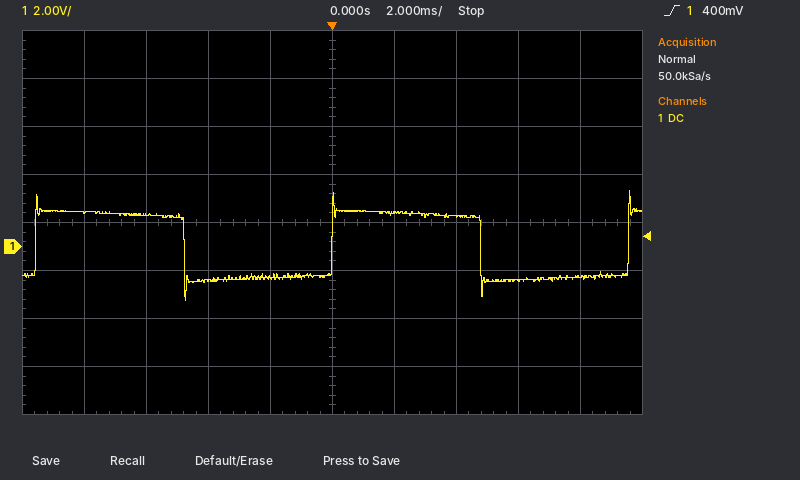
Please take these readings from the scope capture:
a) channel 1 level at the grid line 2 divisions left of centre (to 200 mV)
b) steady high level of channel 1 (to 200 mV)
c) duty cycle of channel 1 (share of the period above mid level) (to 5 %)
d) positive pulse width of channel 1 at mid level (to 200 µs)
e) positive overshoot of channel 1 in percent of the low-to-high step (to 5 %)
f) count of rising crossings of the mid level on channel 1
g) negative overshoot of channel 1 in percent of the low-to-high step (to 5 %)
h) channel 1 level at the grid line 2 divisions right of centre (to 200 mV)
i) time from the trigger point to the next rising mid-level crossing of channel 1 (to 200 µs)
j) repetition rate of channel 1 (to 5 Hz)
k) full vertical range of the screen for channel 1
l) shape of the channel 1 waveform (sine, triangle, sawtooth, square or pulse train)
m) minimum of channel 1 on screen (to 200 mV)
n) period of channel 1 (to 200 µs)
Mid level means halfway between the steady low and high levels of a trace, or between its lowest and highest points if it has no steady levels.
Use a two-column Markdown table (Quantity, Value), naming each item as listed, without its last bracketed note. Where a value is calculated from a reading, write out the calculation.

| Quantity | Value |
|---|---|
| channel 1 level at the grid line 2 divisions left of centre | -1.4 V |
| steady high level of channel 1 | 1.4 V |
| duty cycle of channel 1 (share of the period above mid level) | 4.8 ms / 9.6 ms ≈ 50 % |
| positive pulse width of channel 1 at mid level | 4.8 ms |
| positive overshoot of channel 1 in percent of the low-to-high step | 35 % |
| count of rising crossings of the mid level on channel 1 | 3 |
| negative overshoot of channel 1 in percent of the low-to-high step | 35 % |
| channel 1 level at the grid line 2 divisions right of centre | 1.2 V |
| time from the trigger point to the next rising mid-level crossing of channel 1 | 9.6 ms |
| repetition rate of channel 1 | 1 / 9.6 ms ≈ 104 Hz, so 105 Hz to the nearest 5 Hz |
| full vertical range of the screen for channel 1 | 16 V |
| shape of the channel 1 waveform | square |
| minimum of channel 1 on screen | -2.2 V |
| period of channel 1 | 9.6 ms |
